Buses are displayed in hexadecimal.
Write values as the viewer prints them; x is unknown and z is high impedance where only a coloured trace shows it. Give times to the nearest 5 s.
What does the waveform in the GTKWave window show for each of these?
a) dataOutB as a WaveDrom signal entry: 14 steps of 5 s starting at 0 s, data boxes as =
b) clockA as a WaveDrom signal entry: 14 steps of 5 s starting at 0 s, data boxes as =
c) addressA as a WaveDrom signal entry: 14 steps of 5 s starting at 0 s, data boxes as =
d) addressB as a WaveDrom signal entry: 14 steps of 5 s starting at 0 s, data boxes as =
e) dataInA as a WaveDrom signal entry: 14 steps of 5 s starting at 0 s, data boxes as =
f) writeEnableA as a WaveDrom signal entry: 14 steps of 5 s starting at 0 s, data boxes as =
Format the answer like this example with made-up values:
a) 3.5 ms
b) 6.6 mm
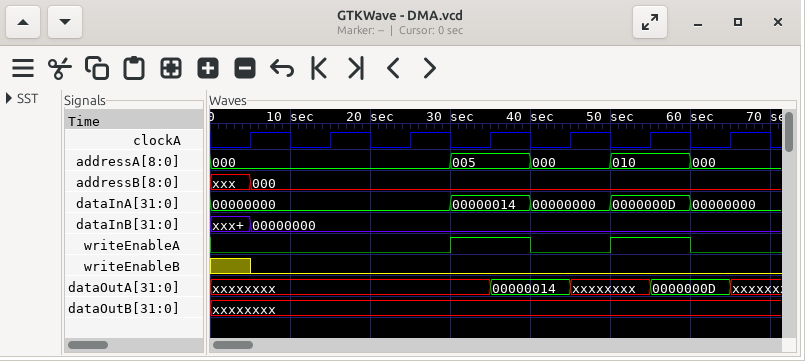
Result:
a) {name: 'dataOutB', wave: 'x.............'}
b) {name: 'clockA', wave: '01010101010101'}
c) {name: 'addressA', wave: '=.....=.=.=.=.', data: '000 005 000 010 000'}
d) {name: 'addressB', wave: 'x=............', data: '000'}
e) {name: 'dataInA', wave: '=.....=.=.=.=.', data: '00000000 00000014 00000000 0000000D 00000000'}
f) {name: 'writeEnableA', wave: '0.....1.0.1.0.'}
